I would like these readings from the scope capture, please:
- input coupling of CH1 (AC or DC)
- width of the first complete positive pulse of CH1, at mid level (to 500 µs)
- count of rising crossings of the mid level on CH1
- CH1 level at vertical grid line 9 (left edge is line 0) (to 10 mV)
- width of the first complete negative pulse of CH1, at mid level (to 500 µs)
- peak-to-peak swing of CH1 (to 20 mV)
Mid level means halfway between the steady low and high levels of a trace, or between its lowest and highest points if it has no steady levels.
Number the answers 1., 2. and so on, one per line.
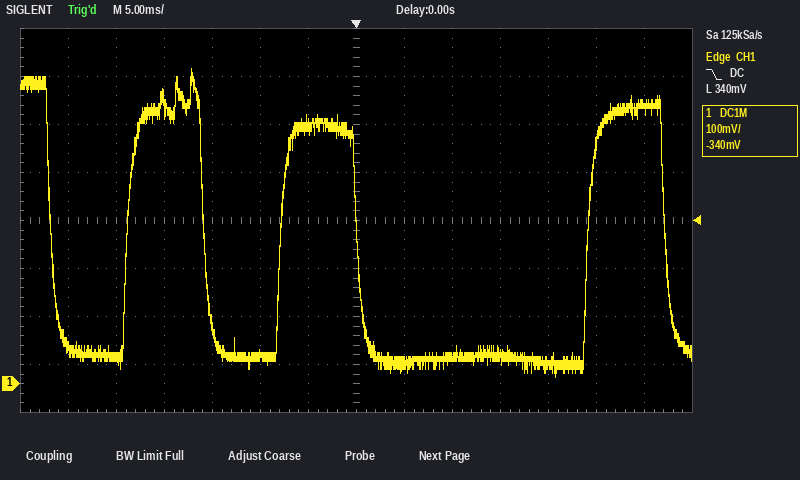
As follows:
1. DC
2. 8.0 ms
3. 3
4. 60 mV
5. 8.0 ms
6. 640 mV
